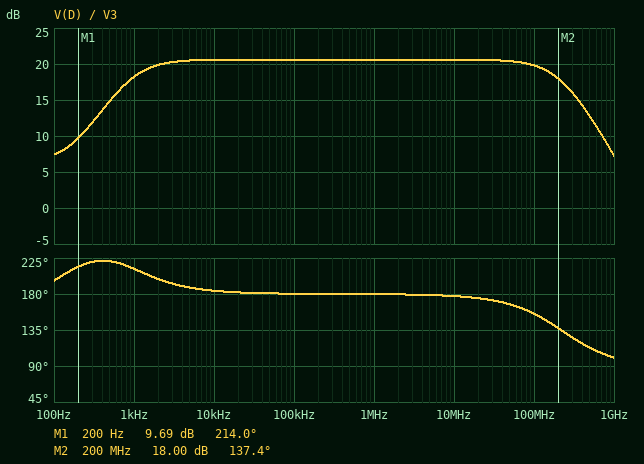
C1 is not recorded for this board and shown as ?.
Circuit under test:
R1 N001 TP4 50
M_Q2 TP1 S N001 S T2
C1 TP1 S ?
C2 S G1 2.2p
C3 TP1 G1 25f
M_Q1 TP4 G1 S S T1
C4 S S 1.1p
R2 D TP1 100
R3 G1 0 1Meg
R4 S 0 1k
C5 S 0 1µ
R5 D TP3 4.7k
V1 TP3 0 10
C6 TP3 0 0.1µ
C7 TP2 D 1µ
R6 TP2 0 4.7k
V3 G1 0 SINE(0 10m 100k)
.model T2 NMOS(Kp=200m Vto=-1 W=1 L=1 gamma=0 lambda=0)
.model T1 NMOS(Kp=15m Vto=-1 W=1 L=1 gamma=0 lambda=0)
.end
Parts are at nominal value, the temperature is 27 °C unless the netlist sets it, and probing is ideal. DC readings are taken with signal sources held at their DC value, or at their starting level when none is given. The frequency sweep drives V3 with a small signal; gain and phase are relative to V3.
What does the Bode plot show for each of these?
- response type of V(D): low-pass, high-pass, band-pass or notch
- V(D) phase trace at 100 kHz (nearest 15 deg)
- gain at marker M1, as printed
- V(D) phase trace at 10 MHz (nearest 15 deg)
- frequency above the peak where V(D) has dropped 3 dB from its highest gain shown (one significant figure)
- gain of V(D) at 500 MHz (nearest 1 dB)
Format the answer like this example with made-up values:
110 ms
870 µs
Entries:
band-pass
180 deg
9.69 dB
180 deg
200 MHz
13 dB
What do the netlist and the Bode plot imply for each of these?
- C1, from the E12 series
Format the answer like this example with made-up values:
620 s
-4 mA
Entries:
270 fF
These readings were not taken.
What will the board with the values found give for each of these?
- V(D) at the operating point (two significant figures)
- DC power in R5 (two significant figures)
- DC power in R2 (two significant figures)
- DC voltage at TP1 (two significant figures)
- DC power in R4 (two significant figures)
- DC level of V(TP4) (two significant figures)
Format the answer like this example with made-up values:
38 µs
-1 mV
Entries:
6.7 V
2.3 mW
48 µW
6.7 V
480 µW
1.6 V
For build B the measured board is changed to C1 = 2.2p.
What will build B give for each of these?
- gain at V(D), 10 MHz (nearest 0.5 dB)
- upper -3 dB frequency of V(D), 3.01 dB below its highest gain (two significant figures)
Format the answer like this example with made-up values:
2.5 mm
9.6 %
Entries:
20.0 dB
29 MHz
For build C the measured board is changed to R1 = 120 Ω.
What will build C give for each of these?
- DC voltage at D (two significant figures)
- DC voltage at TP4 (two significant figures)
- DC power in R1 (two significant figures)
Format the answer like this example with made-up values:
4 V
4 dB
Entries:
6.7 V
1.5 V
58 µW
